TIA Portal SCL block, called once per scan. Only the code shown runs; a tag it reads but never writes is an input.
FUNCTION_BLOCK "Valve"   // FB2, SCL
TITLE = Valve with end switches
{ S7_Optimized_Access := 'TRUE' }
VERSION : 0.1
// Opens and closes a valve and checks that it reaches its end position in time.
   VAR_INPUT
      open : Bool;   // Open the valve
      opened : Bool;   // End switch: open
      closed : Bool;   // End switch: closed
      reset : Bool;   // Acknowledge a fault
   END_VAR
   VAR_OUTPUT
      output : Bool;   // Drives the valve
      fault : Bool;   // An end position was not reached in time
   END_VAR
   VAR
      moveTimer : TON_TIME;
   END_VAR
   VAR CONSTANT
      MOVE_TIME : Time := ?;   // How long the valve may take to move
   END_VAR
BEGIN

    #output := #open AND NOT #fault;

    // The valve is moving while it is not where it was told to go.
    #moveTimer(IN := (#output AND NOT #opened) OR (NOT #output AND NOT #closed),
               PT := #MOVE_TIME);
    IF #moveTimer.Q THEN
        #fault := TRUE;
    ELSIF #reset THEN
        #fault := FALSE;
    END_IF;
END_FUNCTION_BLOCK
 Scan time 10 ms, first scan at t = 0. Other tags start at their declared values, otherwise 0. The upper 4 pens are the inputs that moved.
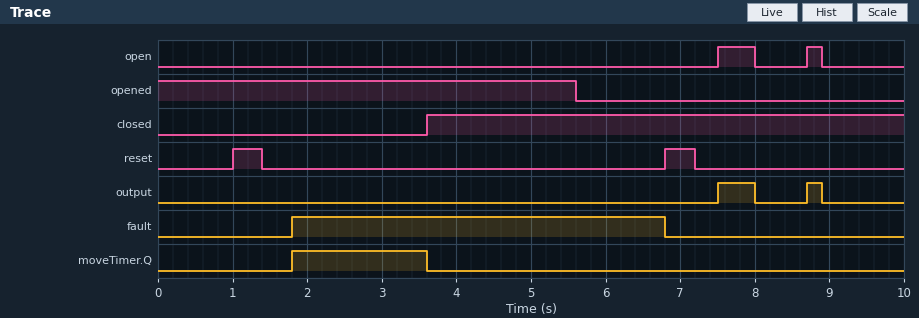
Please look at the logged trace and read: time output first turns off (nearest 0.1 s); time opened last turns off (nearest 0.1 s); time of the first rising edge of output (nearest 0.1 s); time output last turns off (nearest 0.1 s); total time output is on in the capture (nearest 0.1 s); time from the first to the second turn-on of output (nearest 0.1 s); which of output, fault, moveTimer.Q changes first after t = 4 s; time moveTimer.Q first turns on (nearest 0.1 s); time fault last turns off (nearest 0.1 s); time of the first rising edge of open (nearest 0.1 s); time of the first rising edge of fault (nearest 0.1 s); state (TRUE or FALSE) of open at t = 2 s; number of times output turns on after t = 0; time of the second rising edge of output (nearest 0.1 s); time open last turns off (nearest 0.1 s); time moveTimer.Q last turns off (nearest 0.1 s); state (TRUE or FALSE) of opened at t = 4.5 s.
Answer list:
8.0 s
5.6 s
7.5 s
8.9 s
0.7 s
1.2 s
fault
1.8 s
6.8 s
7.5 s
1.8 s
FALSE
2
8.7 s
8.9 s
3.6 s
TRUE
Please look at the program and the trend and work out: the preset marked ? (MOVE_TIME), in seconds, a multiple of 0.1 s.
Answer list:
1.8 s
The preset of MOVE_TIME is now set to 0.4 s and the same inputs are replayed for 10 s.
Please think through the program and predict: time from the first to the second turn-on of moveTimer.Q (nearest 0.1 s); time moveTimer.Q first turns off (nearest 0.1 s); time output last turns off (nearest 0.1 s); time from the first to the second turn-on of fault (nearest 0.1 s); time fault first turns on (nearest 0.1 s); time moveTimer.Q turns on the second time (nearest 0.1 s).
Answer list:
7.5 s
3.6 s
7.9 s
7.5 s
0.4 s
7.9 s
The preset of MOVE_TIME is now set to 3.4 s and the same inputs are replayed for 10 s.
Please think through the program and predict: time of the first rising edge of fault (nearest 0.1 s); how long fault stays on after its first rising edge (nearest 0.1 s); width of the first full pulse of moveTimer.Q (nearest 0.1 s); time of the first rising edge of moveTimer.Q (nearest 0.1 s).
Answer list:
3.4 s
3.4 s
0.2 s
3.4 s
